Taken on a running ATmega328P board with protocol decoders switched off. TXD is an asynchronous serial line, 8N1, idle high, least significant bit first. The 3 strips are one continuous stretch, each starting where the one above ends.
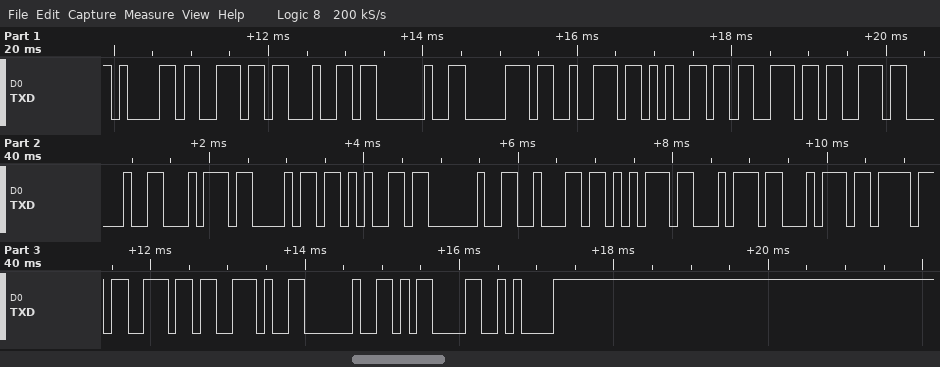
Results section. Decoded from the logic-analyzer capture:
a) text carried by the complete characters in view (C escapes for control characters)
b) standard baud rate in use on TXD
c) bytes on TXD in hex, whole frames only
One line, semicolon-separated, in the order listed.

"and press the button. \r\n"; 9600 baud; 0x61 0x6E 0x64 0x20 0x70 0x72 0x65 0x73 0x73 0x20 0x74 0x68 0x65 0x20 0x62 0x75 0x74 0x74 0x6F 0x6E 0x2E 0x20 0x0D 0x0A
